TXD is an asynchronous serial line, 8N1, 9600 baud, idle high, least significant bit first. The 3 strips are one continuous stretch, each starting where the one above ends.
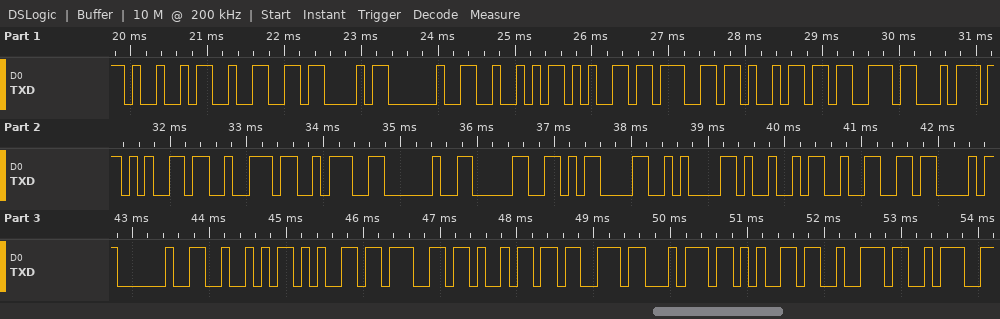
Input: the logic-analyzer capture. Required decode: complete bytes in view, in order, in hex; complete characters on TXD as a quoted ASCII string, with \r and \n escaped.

0x49 0x32 0x43 0x20 0x52 0x65 0x67 0x69 0x73 0x74 0x65 0x72 0x3A 0x20 0x30 0x0D 0x0A 0x49 0x32 0x43 0x20 0x52 0x65 0x67 0x69 0x73 0x74 0x65 0x72 0x3A
"I2C Register: 0\r\nI2C Register:"
